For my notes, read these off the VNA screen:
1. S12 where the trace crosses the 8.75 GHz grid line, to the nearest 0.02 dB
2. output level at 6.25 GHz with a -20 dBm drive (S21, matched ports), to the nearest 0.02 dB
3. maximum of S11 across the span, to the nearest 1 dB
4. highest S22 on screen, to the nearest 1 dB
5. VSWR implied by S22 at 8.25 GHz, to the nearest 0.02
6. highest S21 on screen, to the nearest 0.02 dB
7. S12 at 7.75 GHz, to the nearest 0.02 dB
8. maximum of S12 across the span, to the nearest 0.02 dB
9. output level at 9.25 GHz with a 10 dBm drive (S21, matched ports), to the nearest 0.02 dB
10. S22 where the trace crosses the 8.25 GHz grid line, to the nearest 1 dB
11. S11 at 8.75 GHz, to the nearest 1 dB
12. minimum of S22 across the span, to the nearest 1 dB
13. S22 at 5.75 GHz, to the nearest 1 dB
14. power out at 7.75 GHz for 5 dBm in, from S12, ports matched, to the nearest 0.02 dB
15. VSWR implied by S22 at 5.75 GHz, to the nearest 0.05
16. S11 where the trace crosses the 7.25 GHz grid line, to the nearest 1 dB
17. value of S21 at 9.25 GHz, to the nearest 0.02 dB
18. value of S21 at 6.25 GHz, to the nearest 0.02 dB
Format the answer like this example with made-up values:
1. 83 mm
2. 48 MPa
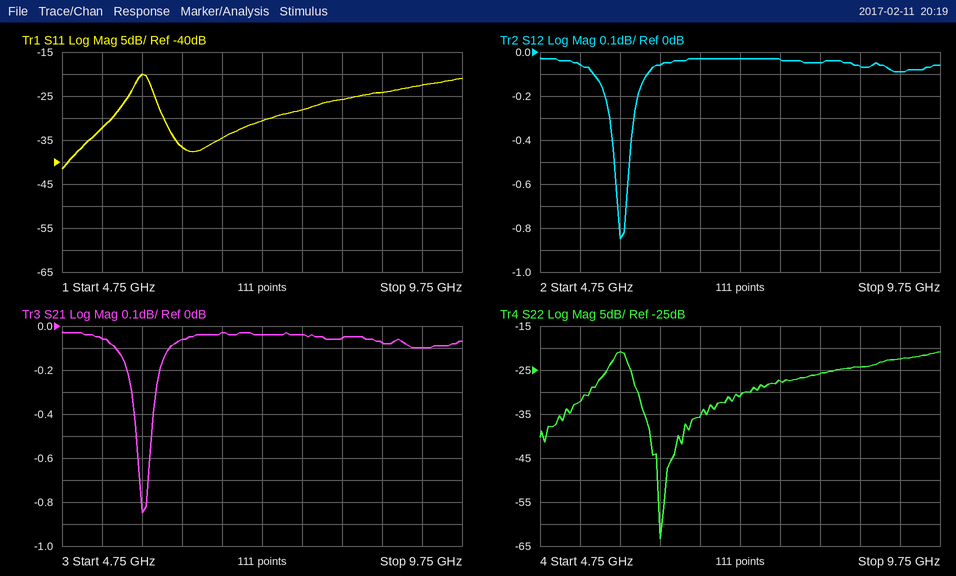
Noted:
1. -0.06 dB
2. -20.06 dBm
3. -20 dB
4. -21 dB
5. 1.10
6. -0.02 dB
7. -0.04 dB
8. -0.02 dB
9. 9.90 dBm
10. -26 dB
11. -24 dB
12. -63 dB
13. -21 dB
14. 4.96 dBm
15. 1.20
16. -31 dB
17. -0.10 dB
18. -0.06 dB
